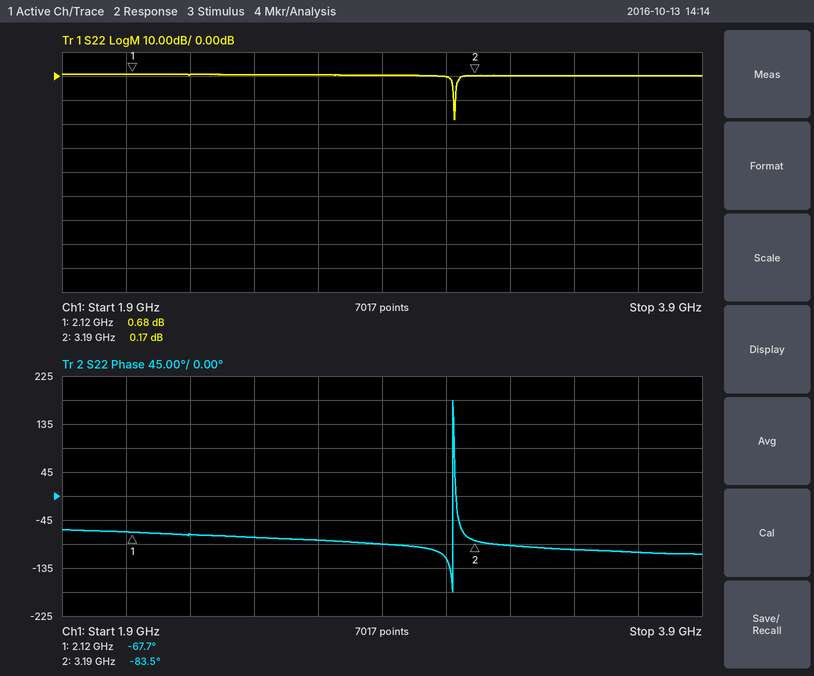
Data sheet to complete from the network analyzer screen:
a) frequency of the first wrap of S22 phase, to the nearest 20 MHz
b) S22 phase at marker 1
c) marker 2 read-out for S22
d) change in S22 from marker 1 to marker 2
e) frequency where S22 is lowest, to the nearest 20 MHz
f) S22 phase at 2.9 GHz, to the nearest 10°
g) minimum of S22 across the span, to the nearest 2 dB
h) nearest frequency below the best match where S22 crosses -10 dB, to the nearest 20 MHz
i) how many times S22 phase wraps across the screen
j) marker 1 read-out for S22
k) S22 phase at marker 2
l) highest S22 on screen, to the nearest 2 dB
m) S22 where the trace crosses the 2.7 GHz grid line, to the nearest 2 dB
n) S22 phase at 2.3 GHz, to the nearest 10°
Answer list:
3.12 GHz
-67.7°
0.17 dB
-0.51 dB
3.12 GHz
-90°
-18 dB
3.12 GHz
1
0.68 dB
-83.5°
0 dB
0 dB
-70°
